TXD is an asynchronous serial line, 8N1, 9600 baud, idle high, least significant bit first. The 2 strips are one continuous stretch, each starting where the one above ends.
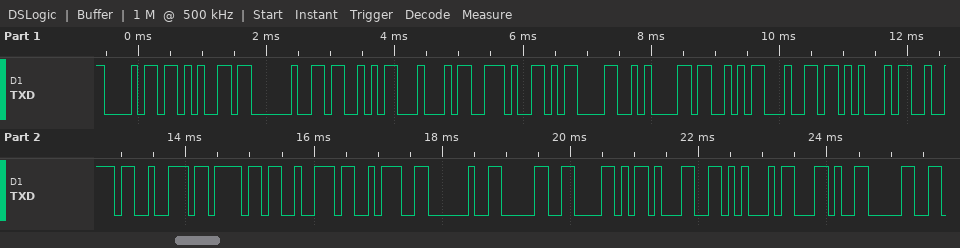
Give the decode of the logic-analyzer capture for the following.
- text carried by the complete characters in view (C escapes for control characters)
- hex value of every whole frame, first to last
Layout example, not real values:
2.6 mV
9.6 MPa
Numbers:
"he SD.\r\nSdError: 0X1E,0"
68 65 20 53 44 2E 0D 0A 53 64 45 72 72 6F 72 3A 20 30 58 31 45 2C 30
